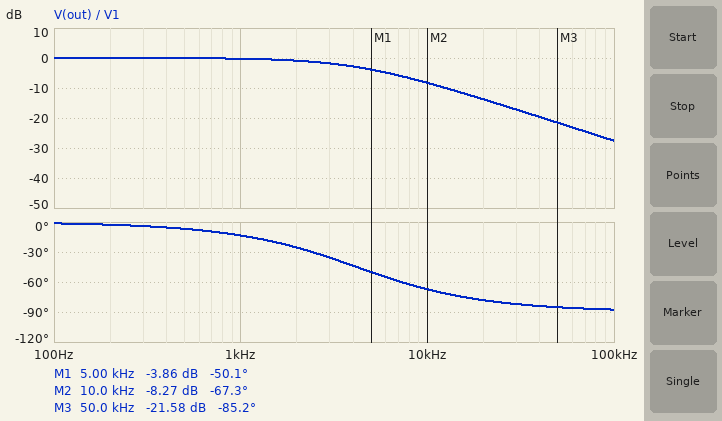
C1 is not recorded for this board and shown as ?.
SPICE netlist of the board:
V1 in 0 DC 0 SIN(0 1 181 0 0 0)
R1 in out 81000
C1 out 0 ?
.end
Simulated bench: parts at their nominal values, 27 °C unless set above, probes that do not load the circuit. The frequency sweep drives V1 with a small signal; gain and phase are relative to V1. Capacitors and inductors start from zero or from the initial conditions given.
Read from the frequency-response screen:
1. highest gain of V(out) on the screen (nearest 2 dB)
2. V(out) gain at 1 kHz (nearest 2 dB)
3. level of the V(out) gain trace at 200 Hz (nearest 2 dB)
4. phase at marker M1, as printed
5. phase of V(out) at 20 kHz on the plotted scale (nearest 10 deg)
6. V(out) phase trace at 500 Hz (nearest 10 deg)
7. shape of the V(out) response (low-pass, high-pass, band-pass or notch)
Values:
0 dB
0 dB
0 dB
-50.1 deg
-80 deg
-10 deg
low-pass
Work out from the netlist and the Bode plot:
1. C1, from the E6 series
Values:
470 pF
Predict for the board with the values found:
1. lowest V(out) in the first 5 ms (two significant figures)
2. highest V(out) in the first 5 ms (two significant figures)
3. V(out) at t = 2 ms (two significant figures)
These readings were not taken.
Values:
-1.0 V
1.0 V
790 mV
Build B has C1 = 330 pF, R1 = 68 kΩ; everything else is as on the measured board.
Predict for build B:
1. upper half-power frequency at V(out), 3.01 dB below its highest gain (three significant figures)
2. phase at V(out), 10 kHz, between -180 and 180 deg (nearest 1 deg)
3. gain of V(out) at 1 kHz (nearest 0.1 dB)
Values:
7.09 kHz
-55 deg
-0.1 dB
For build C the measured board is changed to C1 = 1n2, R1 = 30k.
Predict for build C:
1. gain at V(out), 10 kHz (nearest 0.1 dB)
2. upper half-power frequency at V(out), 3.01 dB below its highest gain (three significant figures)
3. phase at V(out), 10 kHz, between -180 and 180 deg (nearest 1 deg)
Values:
-7.9 dB
4.42 kHz
-66 deg
